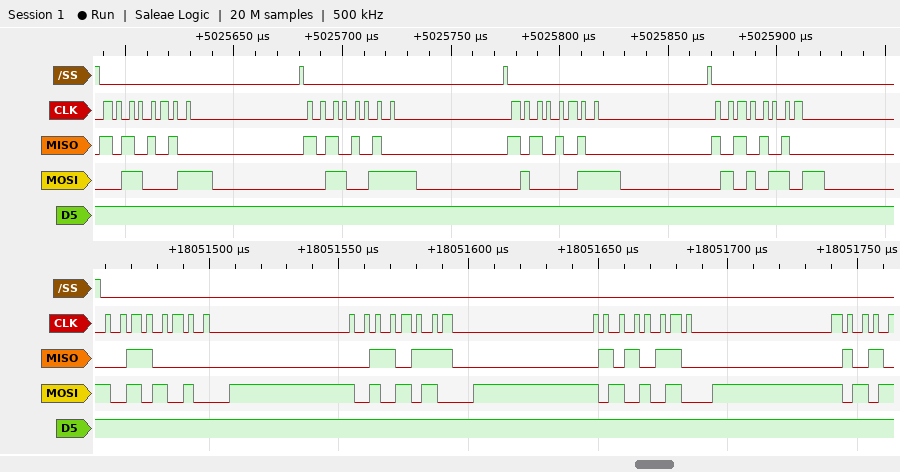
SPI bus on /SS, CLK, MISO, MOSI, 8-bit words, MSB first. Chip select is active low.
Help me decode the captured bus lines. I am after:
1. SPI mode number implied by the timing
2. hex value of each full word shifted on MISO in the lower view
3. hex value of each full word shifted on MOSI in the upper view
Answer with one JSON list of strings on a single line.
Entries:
["0", "30, 37, 56", "31, 33, 43, 56"]
